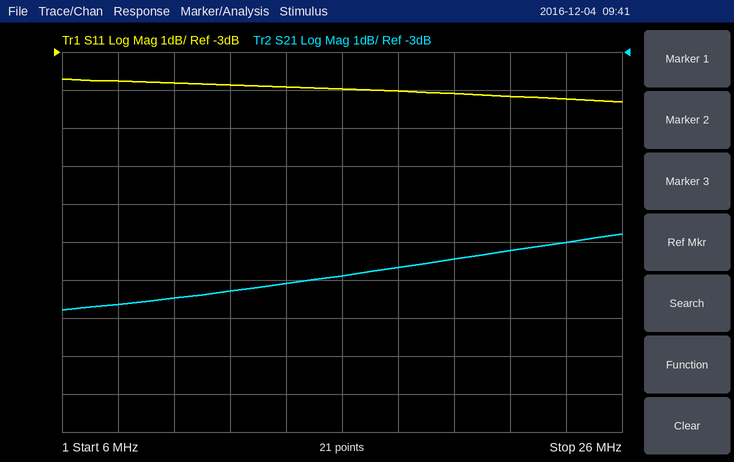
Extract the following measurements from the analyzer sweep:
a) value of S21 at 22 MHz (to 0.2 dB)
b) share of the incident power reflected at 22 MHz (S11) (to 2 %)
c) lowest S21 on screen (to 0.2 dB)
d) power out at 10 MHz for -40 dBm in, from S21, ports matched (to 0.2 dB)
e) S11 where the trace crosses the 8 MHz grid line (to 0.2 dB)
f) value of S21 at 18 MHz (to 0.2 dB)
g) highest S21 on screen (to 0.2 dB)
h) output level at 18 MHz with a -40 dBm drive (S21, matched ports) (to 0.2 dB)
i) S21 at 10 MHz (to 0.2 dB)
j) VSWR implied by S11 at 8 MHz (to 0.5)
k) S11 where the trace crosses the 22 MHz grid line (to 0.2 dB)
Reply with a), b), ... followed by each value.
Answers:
a) -8.2 dB
b) 38 %
c) -9.8 dB
d) -49.4 dBm
e) -3.8 dB
f) -8.6 dB
g) -7.8 dB
h) -48.6 dBm
i) -9.4 dB
j) 4.5
k) -4.2 dB
